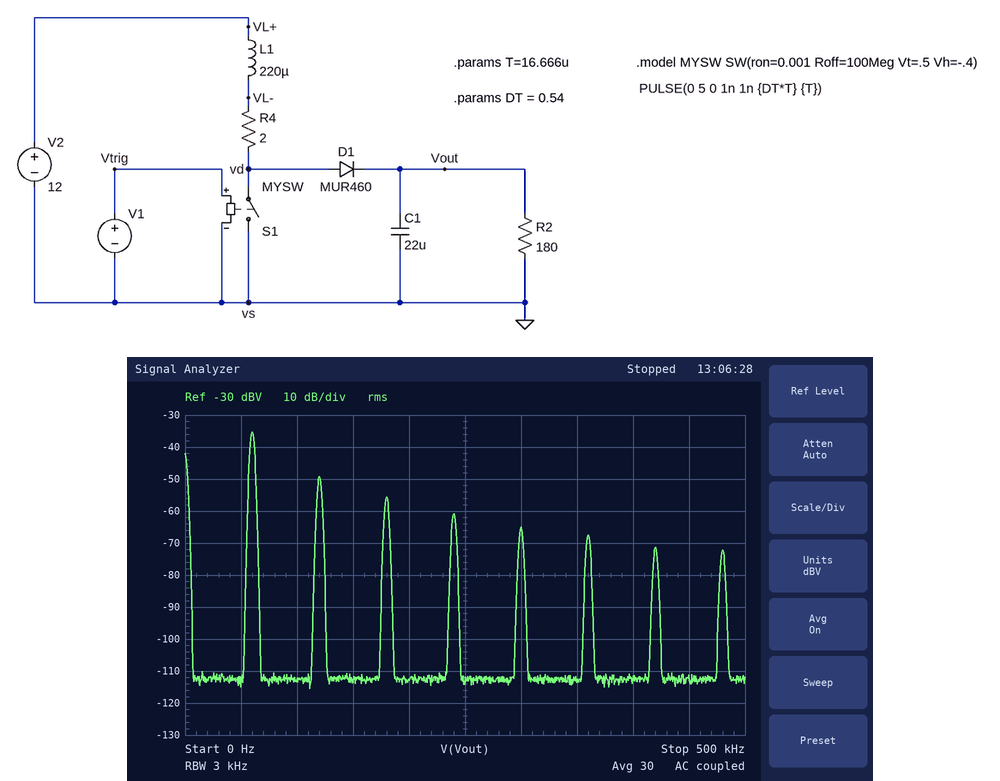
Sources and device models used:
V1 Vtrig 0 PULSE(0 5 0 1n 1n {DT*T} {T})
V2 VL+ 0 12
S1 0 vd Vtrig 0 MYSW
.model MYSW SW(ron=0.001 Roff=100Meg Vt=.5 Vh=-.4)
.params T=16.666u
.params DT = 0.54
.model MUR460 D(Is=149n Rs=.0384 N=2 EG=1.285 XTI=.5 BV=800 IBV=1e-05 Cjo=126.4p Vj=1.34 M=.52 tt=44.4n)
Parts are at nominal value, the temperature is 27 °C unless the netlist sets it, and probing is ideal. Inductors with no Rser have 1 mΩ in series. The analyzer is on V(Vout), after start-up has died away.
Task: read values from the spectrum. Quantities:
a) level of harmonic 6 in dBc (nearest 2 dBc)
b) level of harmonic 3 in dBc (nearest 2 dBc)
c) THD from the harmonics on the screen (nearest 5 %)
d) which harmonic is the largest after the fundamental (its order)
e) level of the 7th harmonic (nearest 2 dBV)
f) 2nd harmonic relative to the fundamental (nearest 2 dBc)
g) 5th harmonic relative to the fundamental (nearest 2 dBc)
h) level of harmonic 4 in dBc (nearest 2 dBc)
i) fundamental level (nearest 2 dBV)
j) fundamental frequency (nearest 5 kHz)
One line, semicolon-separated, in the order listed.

-32 dBc; -20 dBc; 25 %; 2; -72 dBV; -14 dBc; -30 dBc; -26 dBc; -36 dBV; 60 kHz
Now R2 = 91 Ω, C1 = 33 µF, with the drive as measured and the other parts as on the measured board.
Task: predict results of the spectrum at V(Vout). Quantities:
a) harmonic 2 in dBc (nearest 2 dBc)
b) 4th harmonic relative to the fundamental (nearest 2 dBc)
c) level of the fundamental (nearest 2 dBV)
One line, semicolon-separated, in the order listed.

-18 dBc; -28 dBc; -34 dBV
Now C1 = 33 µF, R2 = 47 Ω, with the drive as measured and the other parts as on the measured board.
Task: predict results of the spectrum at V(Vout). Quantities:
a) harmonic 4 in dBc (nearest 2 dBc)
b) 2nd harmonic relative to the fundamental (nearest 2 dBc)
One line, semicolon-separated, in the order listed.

-30 dBc; -22 dBc
